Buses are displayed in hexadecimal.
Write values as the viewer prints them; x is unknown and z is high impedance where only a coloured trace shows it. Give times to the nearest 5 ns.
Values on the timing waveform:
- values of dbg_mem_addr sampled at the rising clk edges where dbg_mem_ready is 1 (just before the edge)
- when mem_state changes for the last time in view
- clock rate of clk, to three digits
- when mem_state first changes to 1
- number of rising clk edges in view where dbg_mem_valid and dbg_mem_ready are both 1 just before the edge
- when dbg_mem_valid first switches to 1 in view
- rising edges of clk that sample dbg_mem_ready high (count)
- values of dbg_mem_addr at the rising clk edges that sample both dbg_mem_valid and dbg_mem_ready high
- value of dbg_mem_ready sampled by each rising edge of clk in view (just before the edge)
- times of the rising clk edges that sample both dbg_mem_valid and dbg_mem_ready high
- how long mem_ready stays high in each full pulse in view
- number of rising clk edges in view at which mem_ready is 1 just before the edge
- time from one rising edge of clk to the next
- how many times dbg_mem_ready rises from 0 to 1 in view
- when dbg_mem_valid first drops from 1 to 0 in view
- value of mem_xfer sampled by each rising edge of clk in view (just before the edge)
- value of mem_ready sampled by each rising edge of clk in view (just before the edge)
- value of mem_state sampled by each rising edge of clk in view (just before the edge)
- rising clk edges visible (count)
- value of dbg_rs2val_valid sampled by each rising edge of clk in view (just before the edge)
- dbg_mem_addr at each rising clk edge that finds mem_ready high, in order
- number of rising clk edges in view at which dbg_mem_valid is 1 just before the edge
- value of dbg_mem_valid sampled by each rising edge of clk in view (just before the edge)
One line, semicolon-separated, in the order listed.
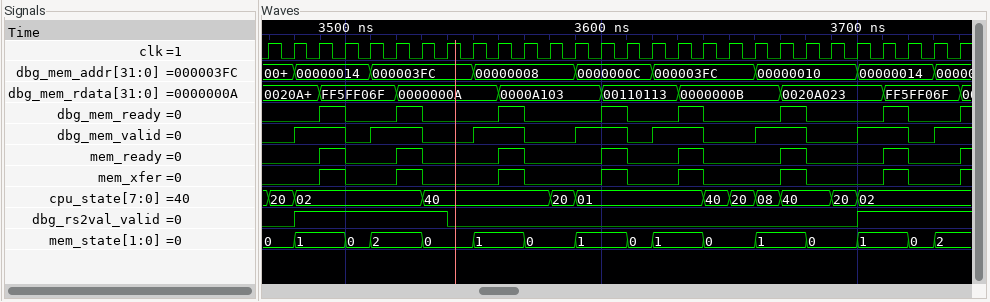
00000014, 000003FC, 00000008, 0000000C, 000003FC, 00000010, 00000014; 3730 ns; 100 MHz; 3480 ns; 7; 3480 ns; 7; 00000014, 000003FC, 00000008, 0000000C, 000003FC, 00000010, 00000014; 0 0 0 1 0 0 1 0 0 0 1 0 0 0 1 0 0 1 0 0 0 1 0 0 0 1 0 0; 3500 ns, 3530 ns, 3570 ns, 3610 ns, 3640 ns, 3680 ns, 3720 ns; 10 ns, 10 ns, 10 ns, 10 ns, 10 ns, 10 ns, 10 ns; 7; 10 ns; 8; 3500 ns; 0 0 0 1 0 0 1 0 0 0 1 0 0 0 1 0 0 1 0 0 0 1 0 0 0 1 0 0; 0 0 0 1 0 0 1 0 0 0 1 0 0 0 1 0 0 1 0 0 0 1 0 0 0 1 0 0; 0, 0, 1, 1, 0, 2, 2, 0, 0, 1, 1, 0, 0, 1, 1, 0, 1, 1, 0, 0, 1, 1, 0, 0, 1, 1, 0, 2; 28; 0 0 1 1 1 1 1 1 0 0 0 0 0 0 0 0 0 0 0 0 0 0 0 0 1 1 1 1; 00000014, 000003FC, 00000008, 0000000C, 000003FC, 00000010, 00000014; 15; 0 0 1 1 0 1 1 0 0 1 1 0 0 1 1 0 1 1 0 0 1 1 0 0 1 1 0 1
